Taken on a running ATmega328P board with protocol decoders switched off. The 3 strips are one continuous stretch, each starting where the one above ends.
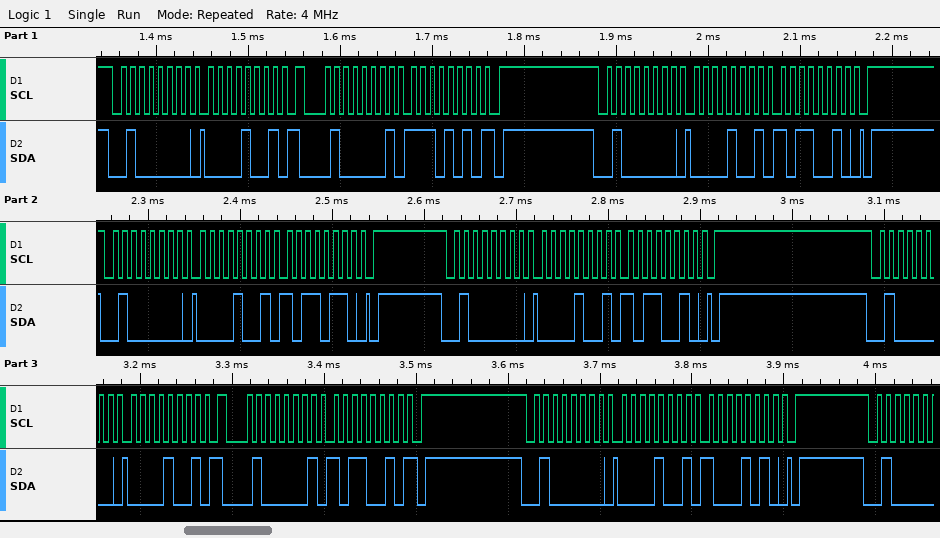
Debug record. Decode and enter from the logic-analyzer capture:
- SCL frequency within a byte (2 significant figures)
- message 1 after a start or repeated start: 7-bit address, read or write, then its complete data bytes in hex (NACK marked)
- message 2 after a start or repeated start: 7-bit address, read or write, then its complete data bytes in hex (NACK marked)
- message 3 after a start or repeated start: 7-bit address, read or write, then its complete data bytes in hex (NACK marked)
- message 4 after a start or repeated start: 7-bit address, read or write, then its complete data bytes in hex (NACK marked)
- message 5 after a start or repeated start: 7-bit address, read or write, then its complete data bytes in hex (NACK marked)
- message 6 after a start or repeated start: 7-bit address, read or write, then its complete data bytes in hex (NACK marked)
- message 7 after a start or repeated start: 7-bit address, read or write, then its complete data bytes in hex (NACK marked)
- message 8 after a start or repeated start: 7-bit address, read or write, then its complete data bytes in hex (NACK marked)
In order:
100 kHz
0x20 write: 09
0x20 read: EA NACK
0x20 write: 09 B2
0x20 write: 09 B6
0x20 write: 09 B2
0x20 write: 09
0x20 read: B2 NACK
0x20 write: 09 8A
